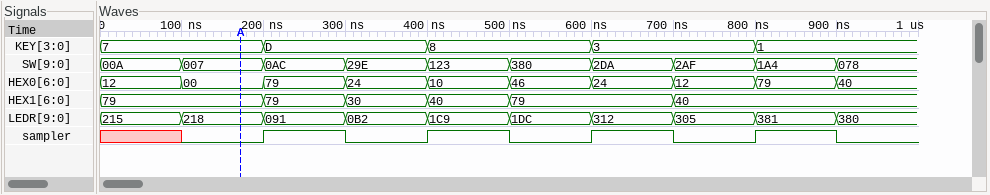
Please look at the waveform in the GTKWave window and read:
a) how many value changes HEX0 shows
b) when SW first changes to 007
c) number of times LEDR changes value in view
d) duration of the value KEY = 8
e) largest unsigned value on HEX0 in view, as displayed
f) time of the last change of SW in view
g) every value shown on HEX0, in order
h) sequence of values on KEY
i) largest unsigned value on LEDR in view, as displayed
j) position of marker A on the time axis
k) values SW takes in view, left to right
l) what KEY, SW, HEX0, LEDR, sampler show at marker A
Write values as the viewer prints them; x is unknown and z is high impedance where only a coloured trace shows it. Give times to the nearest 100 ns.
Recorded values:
9
100 ns
9
200 ns
79
900 ns
12, 00, 79, 24, 10, 46, 24, 12, 79, 40
7, D, 8, 3, 1
381
200 ns
00A, 007, 0AC, 29E, 123, 380, 2DA, 2AF, 1A4, 078
KEY=7, SW=007, HEX0=00, LEDR=218, sampler=0
